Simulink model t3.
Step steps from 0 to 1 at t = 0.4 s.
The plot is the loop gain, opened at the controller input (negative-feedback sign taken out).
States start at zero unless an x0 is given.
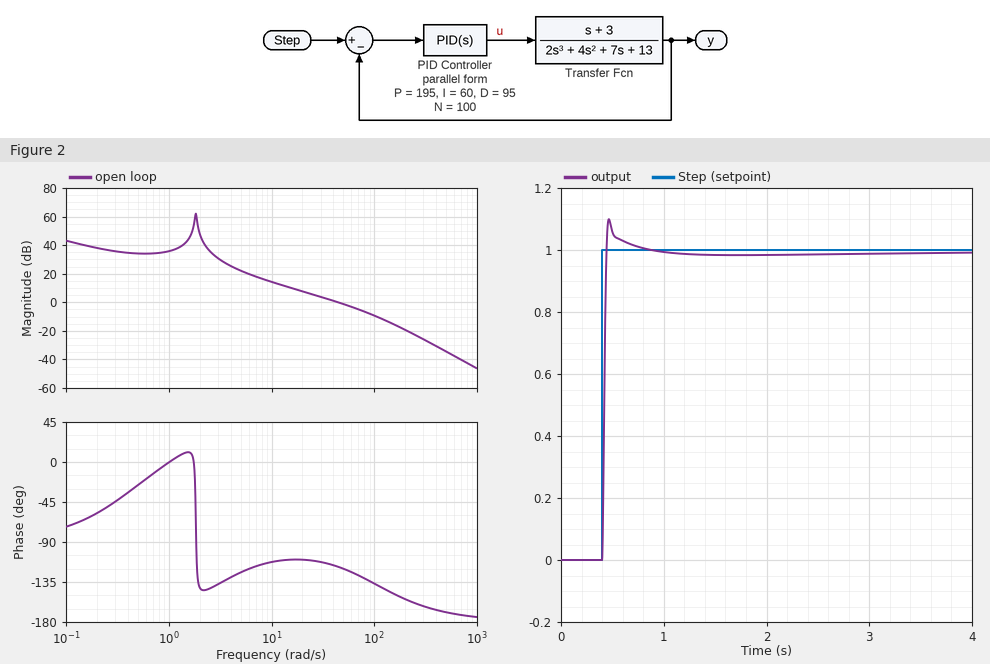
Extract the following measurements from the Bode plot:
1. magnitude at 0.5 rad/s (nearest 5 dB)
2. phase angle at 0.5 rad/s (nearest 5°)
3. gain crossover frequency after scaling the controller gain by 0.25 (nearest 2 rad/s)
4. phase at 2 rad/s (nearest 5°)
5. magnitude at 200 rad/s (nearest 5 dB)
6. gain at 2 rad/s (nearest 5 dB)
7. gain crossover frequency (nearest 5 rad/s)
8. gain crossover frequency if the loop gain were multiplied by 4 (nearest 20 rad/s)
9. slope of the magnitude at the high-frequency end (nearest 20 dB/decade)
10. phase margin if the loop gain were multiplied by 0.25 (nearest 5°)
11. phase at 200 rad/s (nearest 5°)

35 dB
-25°
12 rad/s
-140°
-20 dB
50 dB
45 rad/s
120 rad/s
-40 dB/decade
70°
-155°
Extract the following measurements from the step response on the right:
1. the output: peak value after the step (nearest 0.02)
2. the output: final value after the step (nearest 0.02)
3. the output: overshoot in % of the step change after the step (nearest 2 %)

1.10
1.00
10 %
